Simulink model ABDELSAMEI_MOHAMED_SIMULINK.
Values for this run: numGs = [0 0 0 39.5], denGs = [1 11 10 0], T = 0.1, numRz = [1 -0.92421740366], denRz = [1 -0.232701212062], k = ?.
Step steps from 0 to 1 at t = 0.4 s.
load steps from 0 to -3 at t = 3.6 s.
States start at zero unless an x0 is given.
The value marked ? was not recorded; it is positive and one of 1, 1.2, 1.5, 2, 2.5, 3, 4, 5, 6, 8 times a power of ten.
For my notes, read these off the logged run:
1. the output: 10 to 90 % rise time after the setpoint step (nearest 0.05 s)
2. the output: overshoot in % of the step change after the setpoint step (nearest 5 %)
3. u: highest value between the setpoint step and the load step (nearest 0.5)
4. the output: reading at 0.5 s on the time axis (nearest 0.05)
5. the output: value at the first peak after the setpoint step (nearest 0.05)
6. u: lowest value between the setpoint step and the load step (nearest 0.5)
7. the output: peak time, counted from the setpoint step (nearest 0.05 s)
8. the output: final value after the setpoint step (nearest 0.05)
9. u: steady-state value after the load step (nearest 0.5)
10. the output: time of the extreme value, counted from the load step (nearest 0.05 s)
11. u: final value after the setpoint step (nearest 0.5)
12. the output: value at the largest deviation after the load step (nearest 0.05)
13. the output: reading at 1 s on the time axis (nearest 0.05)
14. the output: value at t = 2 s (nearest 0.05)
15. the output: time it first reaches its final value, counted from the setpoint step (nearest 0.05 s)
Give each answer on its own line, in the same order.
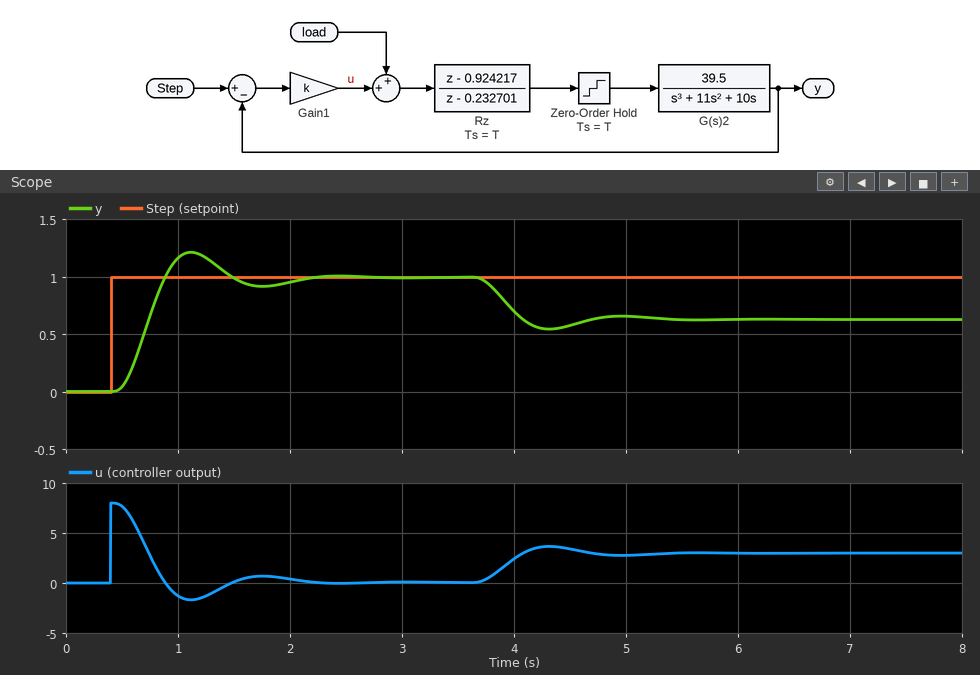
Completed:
0.30 s
20 %
8.0
0.05
1.20
-1.5
0.70 s
1.00
3.0
0.70 s
0.0
0.55
1.15
0.95
0.50 s
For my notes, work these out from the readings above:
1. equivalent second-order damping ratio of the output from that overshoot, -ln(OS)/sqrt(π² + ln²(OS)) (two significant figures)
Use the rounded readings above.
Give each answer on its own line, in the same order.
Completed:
0.46
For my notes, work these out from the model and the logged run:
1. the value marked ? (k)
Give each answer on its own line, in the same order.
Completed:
8
